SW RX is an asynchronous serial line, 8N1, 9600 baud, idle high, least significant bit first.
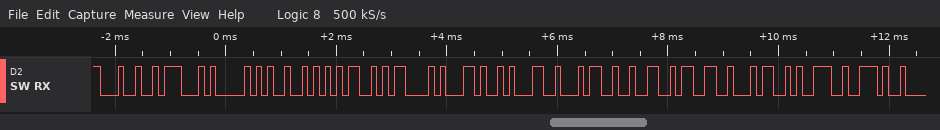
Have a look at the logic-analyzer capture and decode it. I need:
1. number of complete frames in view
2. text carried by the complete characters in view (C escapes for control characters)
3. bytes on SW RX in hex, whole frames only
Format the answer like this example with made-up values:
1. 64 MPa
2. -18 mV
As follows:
1. 14
2. "$GPRMC,142349."
3. 24 47 50 52 4D 43 2C 31 34 32 33 34 39 2E
